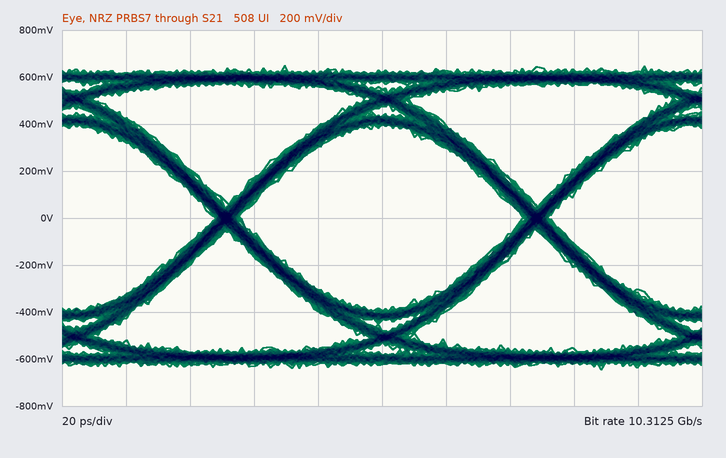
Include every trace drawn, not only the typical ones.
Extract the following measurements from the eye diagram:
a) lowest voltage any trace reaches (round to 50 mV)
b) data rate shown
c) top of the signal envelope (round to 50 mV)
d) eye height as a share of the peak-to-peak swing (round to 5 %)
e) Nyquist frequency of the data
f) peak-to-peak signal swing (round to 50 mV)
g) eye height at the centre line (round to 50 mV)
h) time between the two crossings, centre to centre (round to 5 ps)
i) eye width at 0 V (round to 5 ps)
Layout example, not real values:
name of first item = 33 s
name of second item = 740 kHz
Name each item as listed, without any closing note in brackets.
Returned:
lowest voltage any trace reaches = -650 mV
data rate shown = 10.3125 Gb/s
top of the signal envelope = 650 mV
eye height as a share of the peak-to-peak swing = 60 %
Nyquist frequency of the data = 5.15625 GHz
peak-to-peak signal swing = 1.30 V
eye height at the centre line = 800 mV
time between the two crossings, centre to centre = 95 ps
eye width at 0 V = 90 ps
